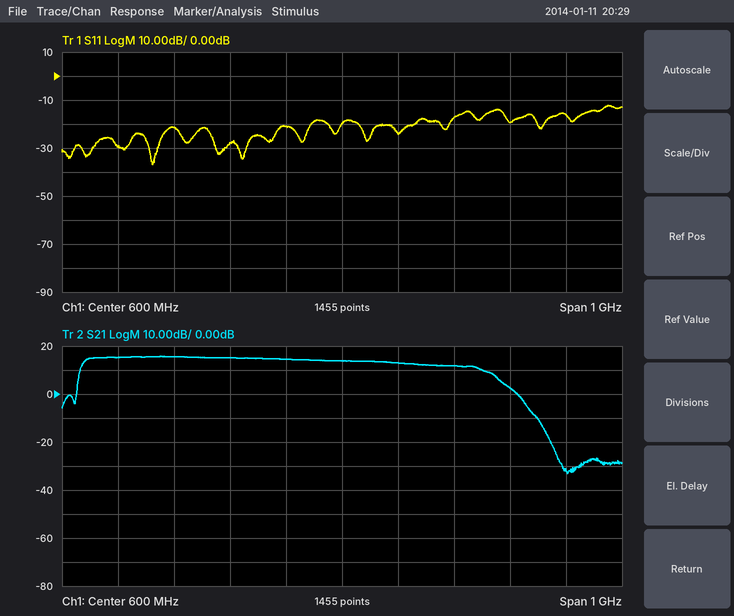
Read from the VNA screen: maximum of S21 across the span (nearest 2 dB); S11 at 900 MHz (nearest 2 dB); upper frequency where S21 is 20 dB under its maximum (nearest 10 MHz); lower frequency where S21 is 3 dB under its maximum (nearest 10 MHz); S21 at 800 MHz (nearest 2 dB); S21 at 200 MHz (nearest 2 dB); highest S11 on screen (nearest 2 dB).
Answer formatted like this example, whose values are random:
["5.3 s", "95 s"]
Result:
["16 dB", "-20 dB", "930 MHz", "140 MHz", "12 dB", "16 dB", "-12 dB"]
